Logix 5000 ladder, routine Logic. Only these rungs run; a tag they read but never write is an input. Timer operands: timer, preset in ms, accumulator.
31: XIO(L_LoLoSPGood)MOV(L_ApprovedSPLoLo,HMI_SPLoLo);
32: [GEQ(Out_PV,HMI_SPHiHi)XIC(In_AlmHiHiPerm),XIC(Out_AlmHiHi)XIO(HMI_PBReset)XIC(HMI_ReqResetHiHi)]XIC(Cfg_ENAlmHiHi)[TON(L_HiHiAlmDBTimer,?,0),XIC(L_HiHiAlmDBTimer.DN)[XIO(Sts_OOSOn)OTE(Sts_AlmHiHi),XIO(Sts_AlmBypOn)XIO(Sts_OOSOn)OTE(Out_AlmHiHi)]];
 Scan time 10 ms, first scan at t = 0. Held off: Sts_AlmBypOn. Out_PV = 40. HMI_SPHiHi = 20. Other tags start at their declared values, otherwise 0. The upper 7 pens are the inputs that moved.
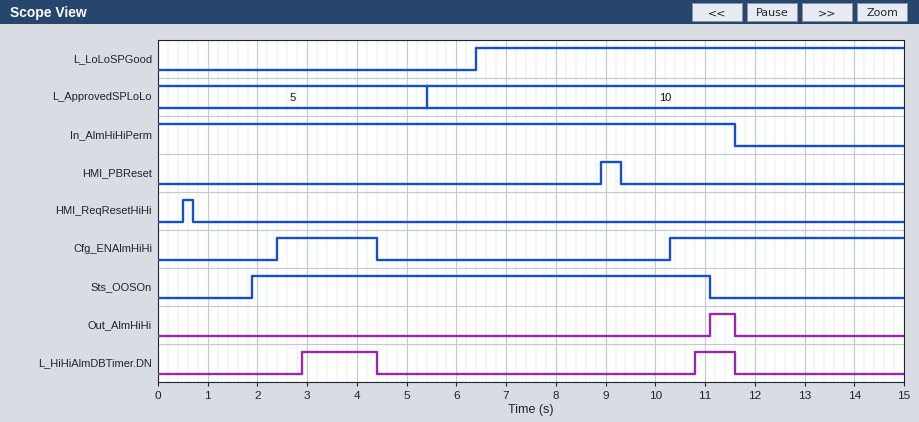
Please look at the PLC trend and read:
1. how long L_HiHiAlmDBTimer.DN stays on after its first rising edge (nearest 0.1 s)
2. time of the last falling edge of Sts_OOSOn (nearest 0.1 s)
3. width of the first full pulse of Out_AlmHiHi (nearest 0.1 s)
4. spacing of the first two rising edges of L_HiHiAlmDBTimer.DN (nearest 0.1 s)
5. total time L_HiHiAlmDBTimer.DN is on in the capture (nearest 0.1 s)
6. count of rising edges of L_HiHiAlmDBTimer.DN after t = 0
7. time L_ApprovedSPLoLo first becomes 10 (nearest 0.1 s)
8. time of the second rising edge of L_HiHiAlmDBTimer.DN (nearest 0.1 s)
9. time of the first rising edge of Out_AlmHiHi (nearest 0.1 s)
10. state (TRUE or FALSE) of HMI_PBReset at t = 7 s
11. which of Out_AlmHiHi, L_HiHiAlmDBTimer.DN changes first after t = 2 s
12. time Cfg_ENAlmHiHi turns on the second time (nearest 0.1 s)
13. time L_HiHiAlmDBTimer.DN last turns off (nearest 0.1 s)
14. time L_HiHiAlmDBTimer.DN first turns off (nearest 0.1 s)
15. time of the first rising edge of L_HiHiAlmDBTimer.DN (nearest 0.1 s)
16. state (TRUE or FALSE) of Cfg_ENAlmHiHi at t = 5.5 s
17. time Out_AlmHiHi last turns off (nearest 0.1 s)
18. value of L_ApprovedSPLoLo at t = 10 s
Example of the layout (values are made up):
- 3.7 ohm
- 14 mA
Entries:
- 1.5 s
- 11.1 s
- 0.5 s
- 7.9 s
- 2.3 s
- 2
- 5.4 s
- 10.8 s
- 11.1 s
- FALSE
- L_HiHiAlmDBTimer.DN
- 10.3 s
- 11.6 s
- 4.4 s
- 2.9 s
- FALSE
- 11.6 s
- 10
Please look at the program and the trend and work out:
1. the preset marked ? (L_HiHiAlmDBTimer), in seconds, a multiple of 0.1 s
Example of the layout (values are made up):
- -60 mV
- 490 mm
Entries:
- 0.5 s
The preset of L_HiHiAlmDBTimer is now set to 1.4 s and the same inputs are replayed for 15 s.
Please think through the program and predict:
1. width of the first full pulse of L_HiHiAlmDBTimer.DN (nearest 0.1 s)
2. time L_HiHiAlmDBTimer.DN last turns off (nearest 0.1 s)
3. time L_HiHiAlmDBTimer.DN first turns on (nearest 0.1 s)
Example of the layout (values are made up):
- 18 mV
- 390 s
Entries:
- 0.6 s
- 4.4 s
- 3.8 s
